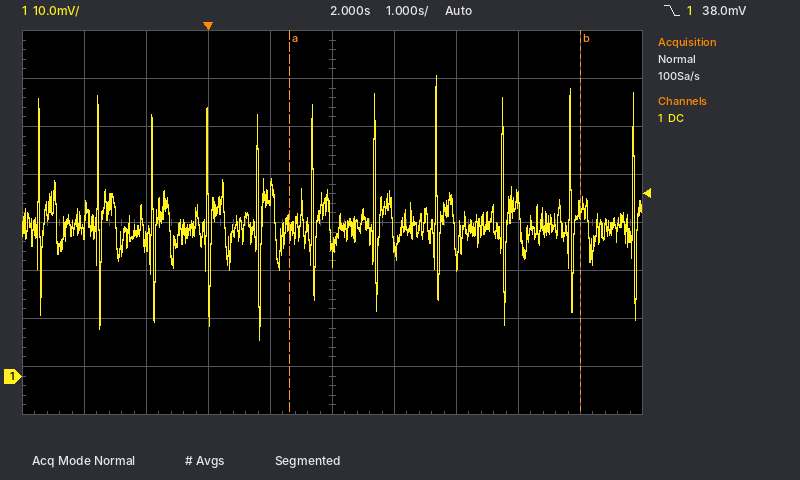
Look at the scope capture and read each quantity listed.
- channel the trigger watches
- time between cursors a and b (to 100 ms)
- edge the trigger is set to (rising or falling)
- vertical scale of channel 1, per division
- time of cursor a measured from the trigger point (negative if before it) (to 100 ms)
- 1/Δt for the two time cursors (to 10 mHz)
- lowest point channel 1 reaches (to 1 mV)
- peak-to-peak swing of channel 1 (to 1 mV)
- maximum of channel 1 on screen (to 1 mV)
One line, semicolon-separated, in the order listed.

channel 1; 4.7 s; falling; 10 mV; +1.3 s; 210 mHz; 8 mV; 55 mV; 63 mV
